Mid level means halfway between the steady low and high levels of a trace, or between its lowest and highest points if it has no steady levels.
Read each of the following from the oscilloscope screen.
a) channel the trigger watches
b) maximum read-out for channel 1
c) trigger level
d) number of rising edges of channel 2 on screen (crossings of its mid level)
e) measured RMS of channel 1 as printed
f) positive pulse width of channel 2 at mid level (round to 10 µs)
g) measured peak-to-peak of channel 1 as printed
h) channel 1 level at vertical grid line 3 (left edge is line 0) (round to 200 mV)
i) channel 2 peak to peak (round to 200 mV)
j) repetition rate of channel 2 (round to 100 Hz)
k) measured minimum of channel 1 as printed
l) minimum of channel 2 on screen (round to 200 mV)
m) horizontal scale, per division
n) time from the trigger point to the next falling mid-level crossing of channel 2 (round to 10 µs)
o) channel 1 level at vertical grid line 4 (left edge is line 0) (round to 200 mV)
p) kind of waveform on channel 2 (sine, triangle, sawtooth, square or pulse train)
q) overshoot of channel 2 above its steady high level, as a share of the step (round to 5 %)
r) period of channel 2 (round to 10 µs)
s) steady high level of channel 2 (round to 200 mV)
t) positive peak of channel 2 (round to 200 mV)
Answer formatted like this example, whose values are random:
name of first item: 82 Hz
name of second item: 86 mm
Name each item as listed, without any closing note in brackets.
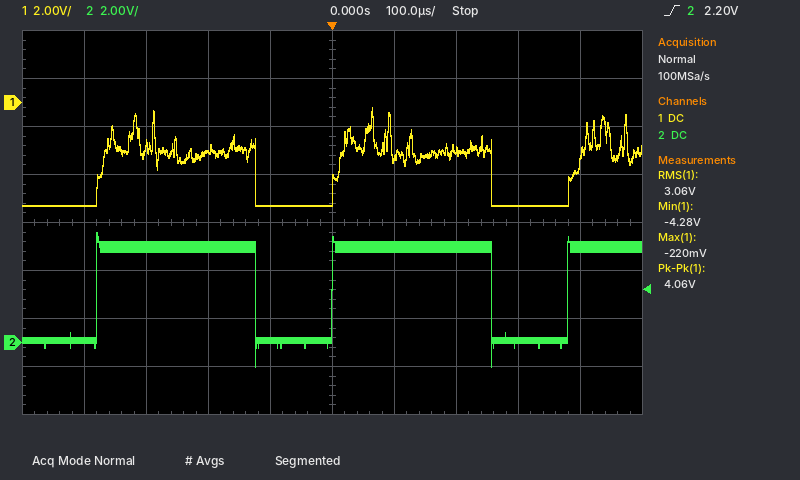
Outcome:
channel the trigger watches: channel 2
maximum read-out for channel 1: -220 mV
trigger level: 2.20 V
number of rising edges of channel 2 on screen: 3
measured RMS of channel 1 as printed: 3.06 V
positive pulse width of channel 2 at mid level: 260 µs
measured peak-to-peak of channel 1 as printed: 4.06 V
channel 1 level at vertical grid line 3 (left edge is line 0): -2.0 V
channel 2 peak to peak: 5.6 V
repetition rate of channel 2: 2.6 kHz
measured minimum of channel 1 as printed: -4.28 V
minimum of channel 2 on screen: -1.0 V
horizontal scale, per division: 100 µs
time from the trigger point to the next falling mid-level crossing of channel 2: 260 µs
channel 1 level at vertical grid line 4 (left edge is line 0): -4.2 V
kind of waveform on channel 2: pulse train
overshoot of channel 2 above its steady high level, as a share of the step: 15 %
period of channel 2: 380 µs
steady high level of channel 2: 4.0 V
positive peak of channel 2: 4.6 V
